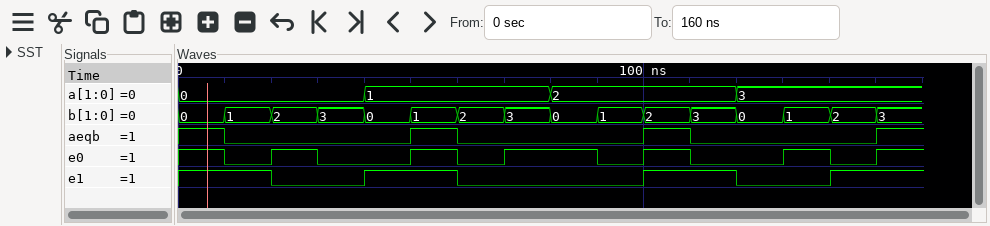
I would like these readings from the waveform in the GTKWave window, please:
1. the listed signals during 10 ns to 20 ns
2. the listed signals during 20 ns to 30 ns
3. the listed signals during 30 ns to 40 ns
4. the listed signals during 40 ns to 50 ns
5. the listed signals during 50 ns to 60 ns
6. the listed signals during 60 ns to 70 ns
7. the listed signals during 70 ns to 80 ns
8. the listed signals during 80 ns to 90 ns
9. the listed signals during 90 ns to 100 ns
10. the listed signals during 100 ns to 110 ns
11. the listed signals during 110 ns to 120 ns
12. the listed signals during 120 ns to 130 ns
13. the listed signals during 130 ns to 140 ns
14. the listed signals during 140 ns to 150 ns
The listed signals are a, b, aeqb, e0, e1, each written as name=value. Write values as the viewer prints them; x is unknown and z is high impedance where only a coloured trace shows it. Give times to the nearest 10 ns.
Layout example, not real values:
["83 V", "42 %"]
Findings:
["a=0, b=1, aeqb=0, e0=0, e1=1", "a=0, b=2, aeqb=0, e0=1, e1=0", "a=0, b=3, aeqb=0, e0=0, e1=0", "a=1, b=0, aeqb=0, e0=0, e1=1", "a=1, b=1, aeqb=1, e0=1, e1=1", "a=1, b=2, aeqb=0, e0=0, e1=0", "a=1, b=3, aeqb=0, e0=1, e1=0", "a=2, b=0, aeqb=0, e0=1, e1=0", "a=2, b=1, aeqb=0, e0=0, e1=0", "a=2, b=2, aeqb=1, e0=1, e1=1", "a=2, b=3, aeqb=0, e0=0, e1=1", "a=3, b=0, aeqb=0, e0=0, e1=0", "a=3, b=1, aeqb=0, e0=1, e1=0", "a=3, b=2, aeqb=0, e0=0, e1=1"]
